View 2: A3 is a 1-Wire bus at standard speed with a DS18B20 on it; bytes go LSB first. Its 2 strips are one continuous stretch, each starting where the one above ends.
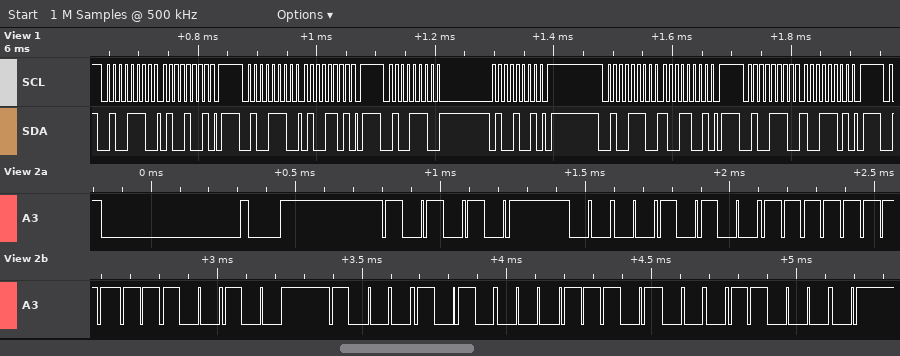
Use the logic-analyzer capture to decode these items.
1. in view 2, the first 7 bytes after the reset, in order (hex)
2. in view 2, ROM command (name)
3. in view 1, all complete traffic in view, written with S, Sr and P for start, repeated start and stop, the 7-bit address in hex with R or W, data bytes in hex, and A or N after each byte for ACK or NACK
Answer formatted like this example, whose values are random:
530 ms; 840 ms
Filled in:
55 28 FF 27 51 B8 18; Match ROM; S 27W A 49 A P S 27W A 4D A P S 27W A 49 A P S 27W A 99 A P S 27W A 9D A P
